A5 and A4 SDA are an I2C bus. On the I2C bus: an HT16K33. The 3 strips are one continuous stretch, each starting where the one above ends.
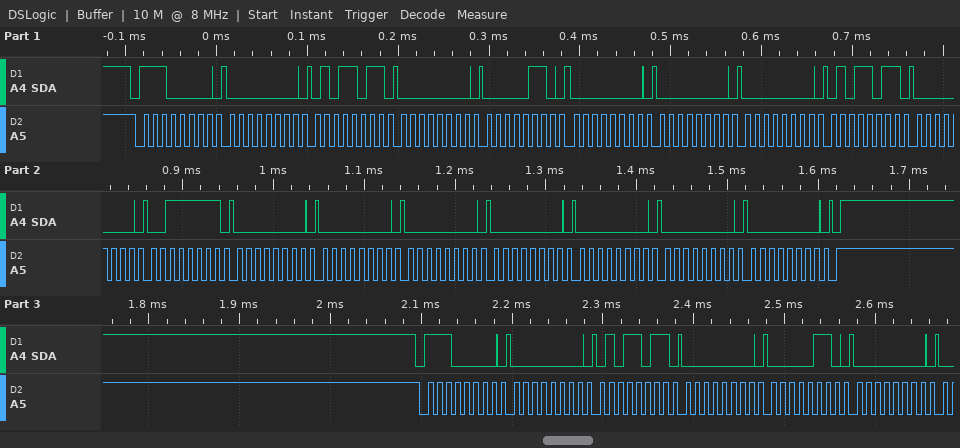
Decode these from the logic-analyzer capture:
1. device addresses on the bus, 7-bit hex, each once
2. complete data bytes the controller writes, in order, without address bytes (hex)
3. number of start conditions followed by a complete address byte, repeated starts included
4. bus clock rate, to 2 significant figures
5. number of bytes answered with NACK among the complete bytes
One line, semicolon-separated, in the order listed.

0x70; 00 5B 00 06 00 00 00 5B 00 3F 00 00 00 00 00 00 00 00 5B 00 06 00; 2; 100 kHz; 0
